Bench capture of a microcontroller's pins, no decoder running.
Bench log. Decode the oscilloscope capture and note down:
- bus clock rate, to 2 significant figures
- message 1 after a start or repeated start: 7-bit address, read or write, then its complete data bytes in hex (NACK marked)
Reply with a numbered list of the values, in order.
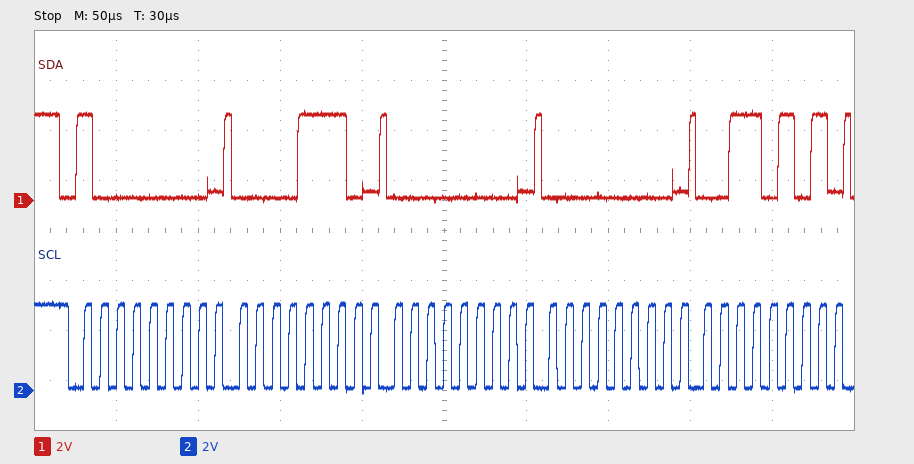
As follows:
1. 100 kHz
2. 0x40 write: 0E 00 00 35
